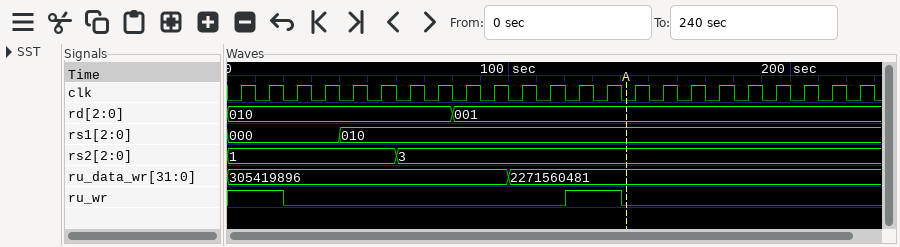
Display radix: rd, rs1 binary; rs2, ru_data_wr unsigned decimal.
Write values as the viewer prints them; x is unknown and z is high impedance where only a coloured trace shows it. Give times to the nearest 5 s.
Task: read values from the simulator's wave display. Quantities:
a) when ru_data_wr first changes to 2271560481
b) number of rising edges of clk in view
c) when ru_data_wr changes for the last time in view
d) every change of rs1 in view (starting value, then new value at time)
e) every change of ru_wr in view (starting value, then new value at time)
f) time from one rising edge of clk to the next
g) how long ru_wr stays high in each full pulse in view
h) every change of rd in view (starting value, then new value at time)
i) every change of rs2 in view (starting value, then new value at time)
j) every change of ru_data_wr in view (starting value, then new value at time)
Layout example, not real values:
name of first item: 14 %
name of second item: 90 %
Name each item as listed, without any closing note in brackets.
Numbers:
when ru_data_wr first changes to 2271560481: 100 s
number of rising edges of clk in view: 23
when ru_data_wr changes for the last time in view: 100 s
every change of rs1 in view: 000, 010 at 40 s
every change of ru_wr in view: 1, 0 at 20 s, 1 at 120 s, 0 at 140 s
time from one rising edge of clk to the next: 10 s
how long ru_wr stays high in each full pulse in view: 20 s
every change of rd in view: 010, 001 at 80 s
every change of rs2 in view: 1, 3 at 60 s
every change of ru_data_wr in view: 305419896, 2271560481 at 100 s
